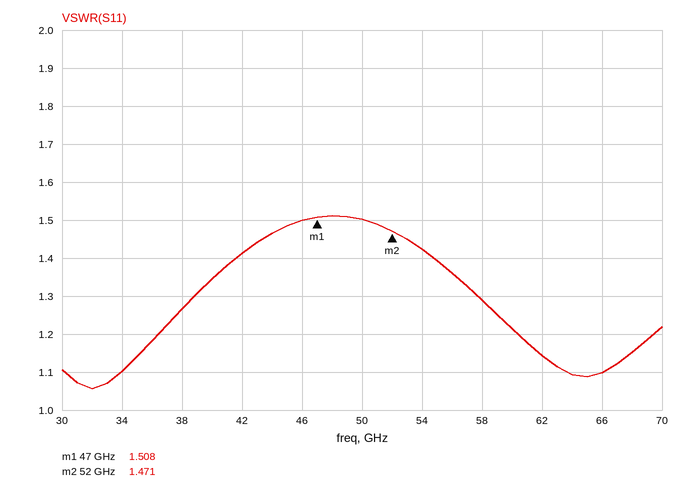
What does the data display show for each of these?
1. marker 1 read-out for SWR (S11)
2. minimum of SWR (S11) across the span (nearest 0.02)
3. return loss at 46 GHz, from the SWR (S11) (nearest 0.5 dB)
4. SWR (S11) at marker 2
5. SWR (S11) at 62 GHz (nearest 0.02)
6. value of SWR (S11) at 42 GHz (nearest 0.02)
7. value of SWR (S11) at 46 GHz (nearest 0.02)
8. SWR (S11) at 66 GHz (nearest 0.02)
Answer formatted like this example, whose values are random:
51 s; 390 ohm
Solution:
1.508; 1.06; 14.0 dB; 1.471; 1.14; 1.42; 1.50; 1.10
